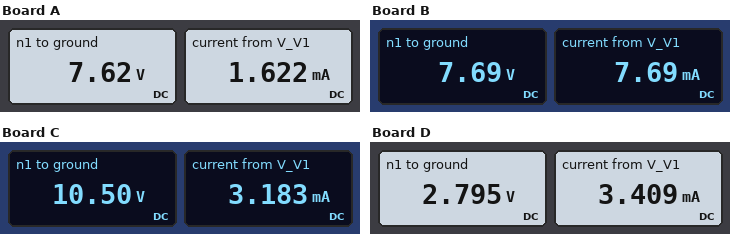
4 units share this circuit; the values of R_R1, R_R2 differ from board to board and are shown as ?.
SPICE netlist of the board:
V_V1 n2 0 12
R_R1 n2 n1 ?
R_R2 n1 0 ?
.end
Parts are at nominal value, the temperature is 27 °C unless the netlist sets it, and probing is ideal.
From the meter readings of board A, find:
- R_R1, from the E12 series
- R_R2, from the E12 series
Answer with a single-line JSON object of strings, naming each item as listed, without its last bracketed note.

{"R_R1, from the E12 series": "2.7 kΩ", "R_R2, from the E12 series": "4.7 kΩ"}
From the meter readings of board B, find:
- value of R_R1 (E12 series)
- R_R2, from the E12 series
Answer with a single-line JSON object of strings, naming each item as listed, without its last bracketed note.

{"value of R_R1": "560 Ω", "R_R2, from the E12 series": "1 kΩ"}
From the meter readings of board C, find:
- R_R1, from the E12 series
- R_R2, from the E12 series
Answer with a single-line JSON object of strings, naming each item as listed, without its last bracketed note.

{"R_R1, from the E12 series": "470 Ω", "R_R2, from the E12 series": "3.3 kΩ"}
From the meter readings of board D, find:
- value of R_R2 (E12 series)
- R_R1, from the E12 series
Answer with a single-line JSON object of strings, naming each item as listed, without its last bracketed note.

{"value of R_R2": "820 Ω", "R_R1, from the E12 series": "2.7 kΩ"}
